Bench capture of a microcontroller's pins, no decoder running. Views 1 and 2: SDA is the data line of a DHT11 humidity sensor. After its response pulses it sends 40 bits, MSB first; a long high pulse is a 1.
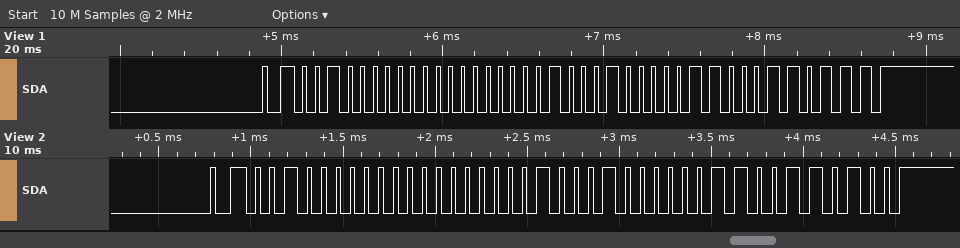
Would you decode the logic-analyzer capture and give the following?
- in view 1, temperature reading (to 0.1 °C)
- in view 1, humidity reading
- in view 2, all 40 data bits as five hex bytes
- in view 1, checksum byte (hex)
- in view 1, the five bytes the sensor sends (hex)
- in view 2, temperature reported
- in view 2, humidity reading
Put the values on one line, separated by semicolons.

17.6 °C; 32 %; 20 00 11 03 34; 0x37; 20 00 11 06 37; 17.3 °C; 32 %
